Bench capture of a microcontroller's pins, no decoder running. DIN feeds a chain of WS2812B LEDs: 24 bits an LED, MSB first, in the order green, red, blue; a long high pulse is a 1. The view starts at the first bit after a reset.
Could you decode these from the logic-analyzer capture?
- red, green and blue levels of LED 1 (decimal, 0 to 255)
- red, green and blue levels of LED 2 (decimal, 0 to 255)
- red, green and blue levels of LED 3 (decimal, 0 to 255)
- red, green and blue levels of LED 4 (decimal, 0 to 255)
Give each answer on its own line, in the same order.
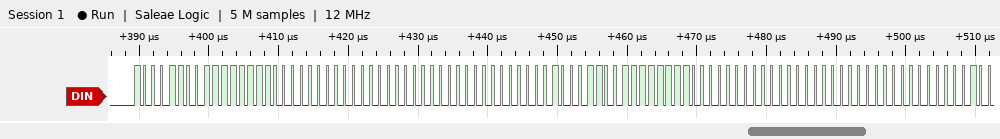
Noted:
255, 140, 0
0, 0, 0
255, 140, 0
0, 0, 0
